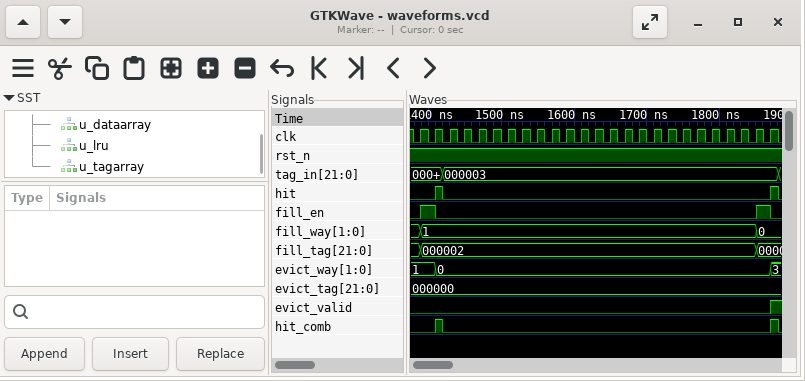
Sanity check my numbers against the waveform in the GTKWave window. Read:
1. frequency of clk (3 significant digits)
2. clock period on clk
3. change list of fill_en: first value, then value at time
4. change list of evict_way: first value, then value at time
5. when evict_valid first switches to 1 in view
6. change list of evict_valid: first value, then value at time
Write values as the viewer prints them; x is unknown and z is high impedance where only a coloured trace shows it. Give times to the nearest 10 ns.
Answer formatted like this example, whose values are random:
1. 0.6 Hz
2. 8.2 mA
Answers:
1. 50.0 MHz
2. 20 ns
3. 0, 1 at 1390 ns, 0 at 1410 ns, 1 at 1850 ns, 0 at 1870 ns
4. 1, 0 at 1410 ns, 3 at 1870 ns
5. 1870 ns
6. 0, 1 at 1870 ns
